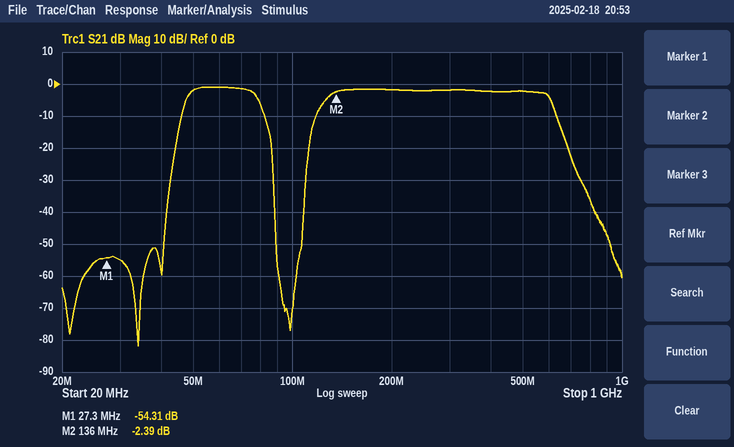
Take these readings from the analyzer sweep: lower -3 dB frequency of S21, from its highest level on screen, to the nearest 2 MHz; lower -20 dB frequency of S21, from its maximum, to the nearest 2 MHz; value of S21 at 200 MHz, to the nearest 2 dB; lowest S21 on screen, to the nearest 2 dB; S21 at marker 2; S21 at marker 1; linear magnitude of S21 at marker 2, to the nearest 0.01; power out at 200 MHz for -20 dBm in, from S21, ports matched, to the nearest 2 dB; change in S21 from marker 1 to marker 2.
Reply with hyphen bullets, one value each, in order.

- 48 MHz
- 44 MHz
- -2 dB
- -82 dB
- -2.39 dB
- -54.31 dB
- 0.76
- -22 dBm
- 51.92 dB
